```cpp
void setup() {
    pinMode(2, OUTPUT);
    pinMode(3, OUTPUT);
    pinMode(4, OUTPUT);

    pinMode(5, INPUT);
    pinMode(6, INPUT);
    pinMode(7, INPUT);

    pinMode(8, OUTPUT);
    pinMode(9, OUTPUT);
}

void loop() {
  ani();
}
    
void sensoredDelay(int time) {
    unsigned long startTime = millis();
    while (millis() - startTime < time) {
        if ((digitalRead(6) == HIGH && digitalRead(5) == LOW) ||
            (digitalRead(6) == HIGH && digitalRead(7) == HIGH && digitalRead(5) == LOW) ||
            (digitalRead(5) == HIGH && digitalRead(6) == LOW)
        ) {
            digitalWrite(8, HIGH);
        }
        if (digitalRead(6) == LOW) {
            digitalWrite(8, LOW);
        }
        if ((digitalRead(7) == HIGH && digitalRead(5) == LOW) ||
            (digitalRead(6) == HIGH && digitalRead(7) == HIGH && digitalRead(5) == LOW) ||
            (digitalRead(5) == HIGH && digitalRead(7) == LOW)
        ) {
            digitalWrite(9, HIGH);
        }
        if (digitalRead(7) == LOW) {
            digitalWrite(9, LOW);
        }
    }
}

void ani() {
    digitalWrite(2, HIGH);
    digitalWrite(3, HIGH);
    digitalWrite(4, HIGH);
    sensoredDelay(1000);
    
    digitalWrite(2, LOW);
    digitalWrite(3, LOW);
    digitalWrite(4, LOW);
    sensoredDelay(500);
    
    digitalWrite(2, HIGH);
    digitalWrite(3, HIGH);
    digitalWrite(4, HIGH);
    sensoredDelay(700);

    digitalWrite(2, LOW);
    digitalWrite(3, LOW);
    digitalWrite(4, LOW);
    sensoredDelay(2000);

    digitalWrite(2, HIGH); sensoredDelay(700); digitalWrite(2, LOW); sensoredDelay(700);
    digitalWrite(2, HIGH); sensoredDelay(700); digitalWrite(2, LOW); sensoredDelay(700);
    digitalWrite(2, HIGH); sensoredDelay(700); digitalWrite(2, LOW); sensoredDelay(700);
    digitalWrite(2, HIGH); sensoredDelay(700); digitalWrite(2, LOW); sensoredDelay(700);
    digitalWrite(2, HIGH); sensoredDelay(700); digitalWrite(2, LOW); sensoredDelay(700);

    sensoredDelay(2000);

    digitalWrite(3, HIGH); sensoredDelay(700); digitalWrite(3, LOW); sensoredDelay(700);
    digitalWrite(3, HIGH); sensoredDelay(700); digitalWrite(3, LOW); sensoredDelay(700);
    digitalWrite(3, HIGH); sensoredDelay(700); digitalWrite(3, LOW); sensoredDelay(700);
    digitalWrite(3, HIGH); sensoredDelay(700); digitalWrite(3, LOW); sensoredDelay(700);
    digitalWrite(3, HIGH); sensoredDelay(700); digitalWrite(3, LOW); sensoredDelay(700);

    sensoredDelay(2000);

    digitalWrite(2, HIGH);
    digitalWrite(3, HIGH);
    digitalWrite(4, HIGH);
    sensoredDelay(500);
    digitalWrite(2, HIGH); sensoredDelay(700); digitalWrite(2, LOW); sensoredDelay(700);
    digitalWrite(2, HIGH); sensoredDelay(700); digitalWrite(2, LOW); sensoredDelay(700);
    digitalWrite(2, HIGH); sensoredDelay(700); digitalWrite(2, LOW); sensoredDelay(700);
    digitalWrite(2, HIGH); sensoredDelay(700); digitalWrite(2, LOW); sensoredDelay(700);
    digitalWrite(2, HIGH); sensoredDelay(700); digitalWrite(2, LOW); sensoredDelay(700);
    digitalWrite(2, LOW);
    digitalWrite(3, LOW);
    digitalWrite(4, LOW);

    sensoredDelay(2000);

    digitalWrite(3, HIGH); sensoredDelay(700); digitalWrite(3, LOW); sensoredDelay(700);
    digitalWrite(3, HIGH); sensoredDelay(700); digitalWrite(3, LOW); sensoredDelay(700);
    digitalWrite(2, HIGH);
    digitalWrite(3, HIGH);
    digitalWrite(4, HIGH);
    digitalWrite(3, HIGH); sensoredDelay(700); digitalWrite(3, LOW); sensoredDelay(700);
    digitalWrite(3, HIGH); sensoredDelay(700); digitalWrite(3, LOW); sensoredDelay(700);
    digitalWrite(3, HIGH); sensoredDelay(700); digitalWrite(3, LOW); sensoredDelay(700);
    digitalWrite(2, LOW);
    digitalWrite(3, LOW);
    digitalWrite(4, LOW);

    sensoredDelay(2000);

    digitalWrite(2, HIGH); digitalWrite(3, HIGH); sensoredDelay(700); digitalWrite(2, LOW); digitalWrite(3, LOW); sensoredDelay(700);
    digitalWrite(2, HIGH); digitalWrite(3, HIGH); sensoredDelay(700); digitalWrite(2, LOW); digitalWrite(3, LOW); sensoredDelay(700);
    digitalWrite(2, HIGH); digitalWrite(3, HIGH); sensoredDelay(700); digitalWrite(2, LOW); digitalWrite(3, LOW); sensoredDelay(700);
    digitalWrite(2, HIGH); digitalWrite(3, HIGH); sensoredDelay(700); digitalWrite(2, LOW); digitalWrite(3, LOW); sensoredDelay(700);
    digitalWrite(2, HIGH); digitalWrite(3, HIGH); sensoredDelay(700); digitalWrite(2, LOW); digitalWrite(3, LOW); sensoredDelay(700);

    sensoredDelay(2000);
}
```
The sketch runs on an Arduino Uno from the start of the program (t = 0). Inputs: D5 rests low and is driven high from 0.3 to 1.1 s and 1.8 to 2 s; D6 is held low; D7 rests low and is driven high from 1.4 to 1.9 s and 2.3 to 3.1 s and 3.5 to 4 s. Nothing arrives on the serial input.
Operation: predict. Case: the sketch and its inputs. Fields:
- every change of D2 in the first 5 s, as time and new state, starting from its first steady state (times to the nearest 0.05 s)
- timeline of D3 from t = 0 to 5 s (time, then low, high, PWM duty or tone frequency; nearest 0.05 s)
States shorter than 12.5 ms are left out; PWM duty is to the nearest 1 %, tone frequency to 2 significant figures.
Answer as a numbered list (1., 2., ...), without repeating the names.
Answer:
1. 0 s high; 1 s low; 1.5 s high; 2.2 s low; 4.2 s high; 4.9 s low
2. 0 s high; 1 s low; 1.5 s high; 2.2 s low
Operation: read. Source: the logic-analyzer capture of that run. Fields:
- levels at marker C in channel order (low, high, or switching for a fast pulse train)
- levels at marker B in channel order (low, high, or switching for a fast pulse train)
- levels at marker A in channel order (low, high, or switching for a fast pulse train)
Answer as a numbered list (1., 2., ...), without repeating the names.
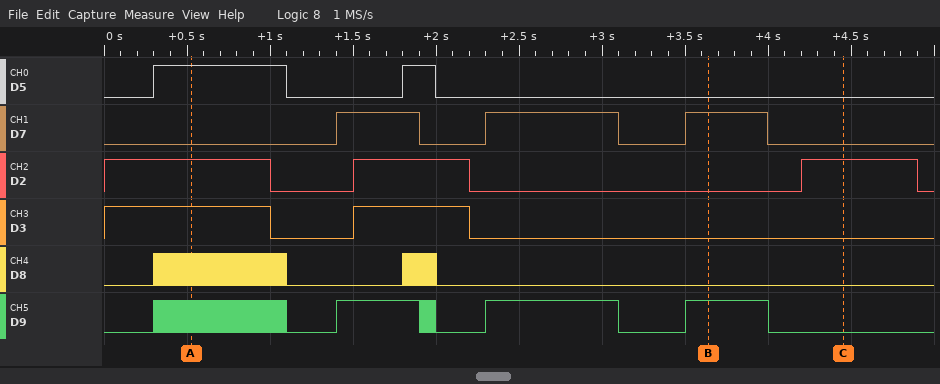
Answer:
1. D5 low, D7 low, D2 high, D3 low, D8 low, D9 low
2. D5 low, D7 high, D2 low, D3 low, D8 low, D9 high
3. D5 high, D7 low, D2 high, D3 high, D8 switching, D9 switching
